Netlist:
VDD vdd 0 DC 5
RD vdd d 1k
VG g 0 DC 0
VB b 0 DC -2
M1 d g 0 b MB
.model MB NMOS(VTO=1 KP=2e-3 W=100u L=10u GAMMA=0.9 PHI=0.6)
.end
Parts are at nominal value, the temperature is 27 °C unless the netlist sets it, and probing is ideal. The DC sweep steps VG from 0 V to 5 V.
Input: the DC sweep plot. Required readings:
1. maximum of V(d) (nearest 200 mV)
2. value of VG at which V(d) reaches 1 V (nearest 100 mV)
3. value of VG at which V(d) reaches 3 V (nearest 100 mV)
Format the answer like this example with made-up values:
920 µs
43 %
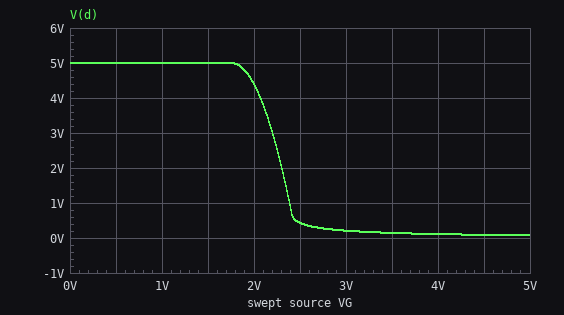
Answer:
5.0 V
2.4 V
2.2 V
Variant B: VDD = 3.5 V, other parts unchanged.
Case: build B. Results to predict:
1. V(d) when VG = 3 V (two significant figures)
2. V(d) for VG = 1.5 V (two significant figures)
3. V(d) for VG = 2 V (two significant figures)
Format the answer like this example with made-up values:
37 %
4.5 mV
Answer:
140 mV
3.5 V
2.9 V
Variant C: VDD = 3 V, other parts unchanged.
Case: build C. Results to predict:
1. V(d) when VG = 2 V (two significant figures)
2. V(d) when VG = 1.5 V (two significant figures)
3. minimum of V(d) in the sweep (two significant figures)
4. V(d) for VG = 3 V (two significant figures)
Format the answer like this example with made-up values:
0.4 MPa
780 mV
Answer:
2.4 V
3.0 V
46 mV
120 mV
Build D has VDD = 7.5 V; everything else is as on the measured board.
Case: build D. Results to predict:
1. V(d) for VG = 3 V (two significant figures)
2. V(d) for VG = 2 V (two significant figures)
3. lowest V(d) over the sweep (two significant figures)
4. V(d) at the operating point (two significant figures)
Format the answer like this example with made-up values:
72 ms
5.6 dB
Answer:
330 mV
6.9 V
120 mV
7.5 V
